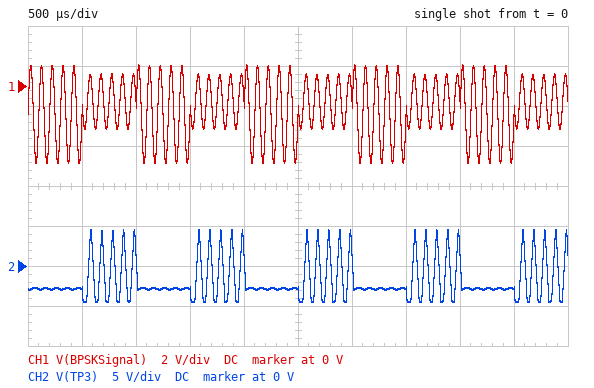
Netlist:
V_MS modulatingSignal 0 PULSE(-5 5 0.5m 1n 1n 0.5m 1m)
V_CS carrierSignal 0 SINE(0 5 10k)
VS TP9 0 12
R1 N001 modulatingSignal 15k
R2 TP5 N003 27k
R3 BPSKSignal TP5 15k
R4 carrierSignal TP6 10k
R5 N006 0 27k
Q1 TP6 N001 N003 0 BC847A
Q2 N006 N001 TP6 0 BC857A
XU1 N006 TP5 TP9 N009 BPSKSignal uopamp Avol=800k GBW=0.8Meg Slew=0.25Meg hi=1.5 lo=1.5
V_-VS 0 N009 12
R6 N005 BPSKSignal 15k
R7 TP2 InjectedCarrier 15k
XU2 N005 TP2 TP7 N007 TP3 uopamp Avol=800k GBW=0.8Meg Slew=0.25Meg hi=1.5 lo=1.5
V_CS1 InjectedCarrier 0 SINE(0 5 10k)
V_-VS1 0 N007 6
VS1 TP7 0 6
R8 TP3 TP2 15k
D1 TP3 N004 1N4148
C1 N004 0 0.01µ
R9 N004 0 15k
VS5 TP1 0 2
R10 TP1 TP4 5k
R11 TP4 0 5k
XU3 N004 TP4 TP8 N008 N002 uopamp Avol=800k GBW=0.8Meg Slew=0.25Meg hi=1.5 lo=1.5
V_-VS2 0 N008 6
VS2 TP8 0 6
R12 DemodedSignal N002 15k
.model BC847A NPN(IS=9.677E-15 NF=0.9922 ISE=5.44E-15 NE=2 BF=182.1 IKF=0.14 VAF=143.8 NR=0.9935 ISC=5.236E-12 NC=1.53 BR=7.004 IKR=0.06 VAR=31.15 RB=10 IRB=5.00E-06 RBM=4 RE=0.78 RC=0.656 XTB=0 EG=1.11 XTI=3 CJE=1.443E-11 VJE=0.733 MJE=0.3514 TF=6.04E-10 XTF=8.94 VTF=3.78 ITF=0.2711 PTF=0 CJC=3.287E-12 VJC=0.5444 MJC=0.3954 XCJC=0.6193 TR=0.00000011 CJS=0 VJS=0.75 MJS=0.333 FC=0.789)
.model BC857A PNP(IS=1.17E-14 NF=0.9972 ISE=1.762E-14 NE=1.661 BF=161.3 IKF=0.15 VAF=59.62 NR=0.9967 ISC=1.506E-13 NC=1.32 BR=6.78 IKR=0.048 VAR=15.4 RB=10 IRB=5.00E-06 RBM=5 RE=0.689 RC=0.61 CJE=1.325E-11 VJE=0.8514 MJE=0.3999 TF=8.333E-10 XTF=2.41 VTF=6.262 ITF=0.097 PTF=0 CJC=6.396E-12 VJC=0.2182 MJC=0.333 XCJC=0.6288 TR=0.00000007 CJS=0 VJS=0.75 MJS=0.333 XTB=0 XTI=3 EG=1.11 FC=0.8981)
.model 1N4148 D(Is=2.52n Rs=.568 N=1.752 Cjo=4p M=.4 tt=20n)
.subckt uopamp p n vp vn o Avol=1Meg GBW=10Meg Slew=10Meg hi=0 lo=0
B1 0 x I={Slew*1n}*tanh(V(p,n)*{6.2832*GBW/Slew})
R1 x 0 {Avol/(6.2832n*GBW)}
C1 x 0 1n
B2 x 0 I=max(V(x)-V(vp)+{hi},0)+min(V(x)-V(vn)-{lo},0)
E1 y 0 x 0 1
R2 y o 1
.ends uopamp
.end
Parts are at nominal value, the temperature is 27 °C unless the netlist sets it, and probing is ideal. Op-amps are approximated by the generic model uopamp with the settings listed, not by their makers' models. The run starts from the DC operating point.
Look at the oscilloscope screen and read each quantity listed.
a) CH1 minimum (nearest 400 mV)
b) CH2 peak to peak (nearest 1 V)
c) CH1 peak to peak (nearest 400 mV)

-4.0 V
9 V
4.8 V
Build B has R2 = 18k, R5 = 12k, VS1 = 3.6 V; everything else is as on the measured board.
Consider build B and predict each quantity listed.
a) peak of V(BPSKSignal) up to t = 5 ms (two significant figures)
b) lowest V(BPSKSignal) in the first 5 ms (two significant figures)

840 mV
-3.2 V
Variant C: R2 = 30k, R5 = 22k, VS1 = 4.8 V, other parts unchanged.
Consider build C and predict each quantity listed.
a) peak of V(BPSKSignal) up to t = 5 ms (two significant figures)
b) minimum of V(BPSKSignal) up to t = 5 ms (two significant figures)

990 mV
-3.7 V
